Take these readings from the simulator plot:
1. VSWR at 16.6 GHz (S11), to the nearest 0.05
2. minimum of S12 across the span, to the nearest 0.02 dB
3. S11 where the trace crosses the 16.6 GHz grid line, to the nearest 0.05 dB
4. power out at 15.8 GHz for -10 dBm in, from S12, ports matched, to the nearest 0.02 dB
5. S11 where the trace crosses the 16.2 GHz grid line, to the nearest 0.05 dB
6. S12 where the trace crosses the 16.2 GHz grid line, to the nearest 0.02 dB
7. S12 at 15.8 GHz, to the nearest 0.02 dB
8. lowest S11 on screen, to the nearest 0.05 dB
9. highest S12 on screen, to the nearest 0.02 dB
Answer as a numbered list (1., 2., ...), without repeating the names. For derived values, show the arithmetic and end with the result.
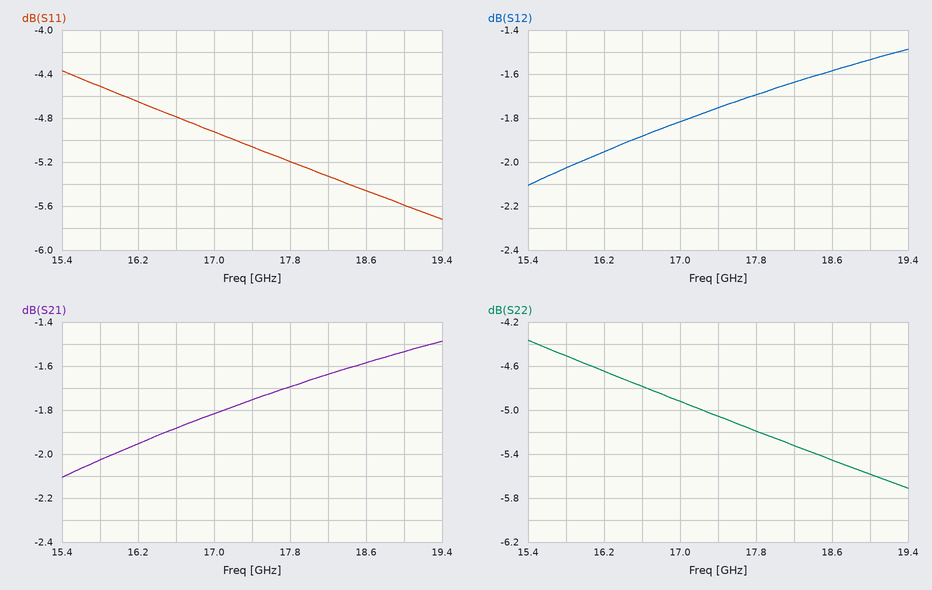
1. |Γ| = 10^(-4.8/20) = 0.5754; VSWR = (1 + 0.5754)/(1 − 0.5754) ≈ 3.71, so 3.70 to the nearest 0.05
2. -2.10 dB
3. -4.80 dB
4. -10 dBm + (-2.02 dB) = -12.02 dBm
5. -4.65 dB
6. -1.96 dB
7. -2.02 dB
8. -5.70 dB
9. -1.48 dB
